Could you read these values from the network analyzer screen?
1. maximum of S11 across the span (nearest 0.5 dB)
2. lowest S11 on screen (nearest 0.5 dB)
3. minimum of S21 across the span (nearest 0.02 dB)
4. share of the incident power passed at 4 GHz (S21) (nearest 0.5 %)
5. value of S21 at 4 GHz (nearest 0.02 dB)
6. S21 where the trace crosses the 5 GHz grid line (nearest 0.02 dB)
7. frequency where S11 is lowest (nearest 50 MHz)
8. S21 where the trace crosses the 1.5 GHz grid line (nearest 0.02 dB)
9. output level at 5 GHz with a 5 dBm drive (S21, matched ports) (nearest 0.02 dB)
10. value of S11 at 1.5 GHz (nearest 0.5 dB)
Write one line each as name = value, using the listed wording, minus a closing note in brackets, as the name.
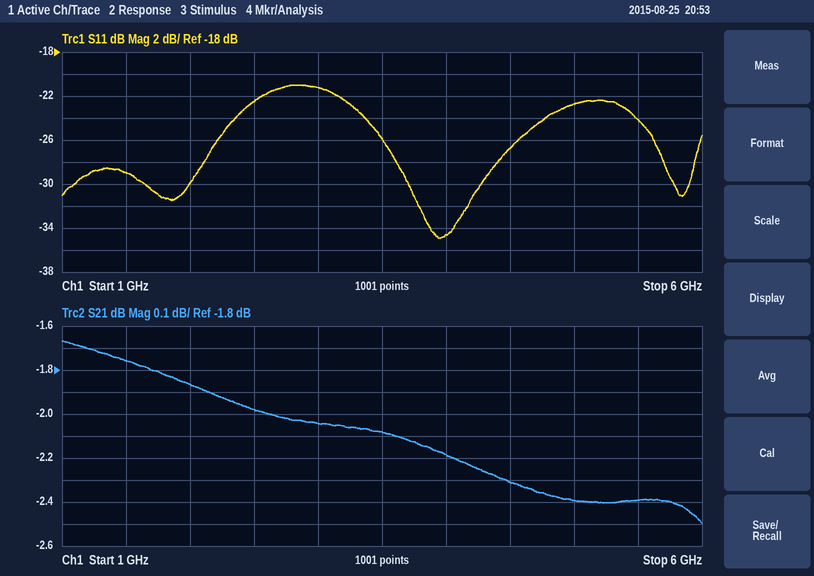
maximum of S11 across the span = -21.0 dB
lowest S11 on screen = -35.0 dB
minimum of S21 across the span = -2.50 dB
share of the incident power passed at 4 GHz (S21) = 60.5 %
value of S21 at 4 GHz = -2.18 dB
S21 where the trace crosses the 5 GHz grid line = -2.40 dB
frequency where S11 is lowest = 3.95 GHz
S21 where the trace crosses the 1.5 GHz grid line = -1.76 dB
output level at 5 GHz with a 5 dBm drive (S21, matched ports) = 2.60 dBm
value of S11 at 1.5 GHz = -29.0 dB
